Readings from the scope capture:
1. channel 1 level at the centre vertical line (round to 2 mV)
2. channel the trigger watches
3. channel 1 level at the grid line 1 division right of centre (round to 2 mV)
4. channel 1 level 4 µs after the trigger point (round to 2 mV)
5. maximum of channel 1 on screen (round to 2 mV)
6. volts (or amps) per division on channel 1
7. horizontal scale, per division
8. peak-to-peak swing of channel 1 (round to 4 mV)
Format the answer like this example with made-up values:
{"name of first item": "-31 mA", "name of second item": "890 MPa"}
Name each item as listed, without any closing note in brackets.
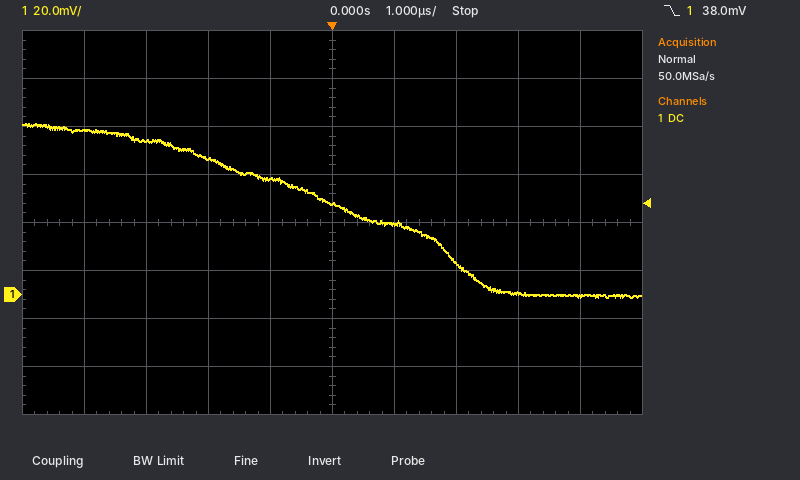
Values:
{"channel 1 level at the centre vertical line": "38 mV", "channel the trigger watches": "channel 1", "channel 1 level at the grid line 1 division right of centre": "30 mV", "channel 1 level 4 µs after the trigger point": "0 mV", "maximum of channel 1 on screen": "72 mV", "volts (or amps) per division on channel 1": "20 mV", "horizontal scale, per division": "1 µs", "peak-to-peak swing of channel 1": "72 mV"}
